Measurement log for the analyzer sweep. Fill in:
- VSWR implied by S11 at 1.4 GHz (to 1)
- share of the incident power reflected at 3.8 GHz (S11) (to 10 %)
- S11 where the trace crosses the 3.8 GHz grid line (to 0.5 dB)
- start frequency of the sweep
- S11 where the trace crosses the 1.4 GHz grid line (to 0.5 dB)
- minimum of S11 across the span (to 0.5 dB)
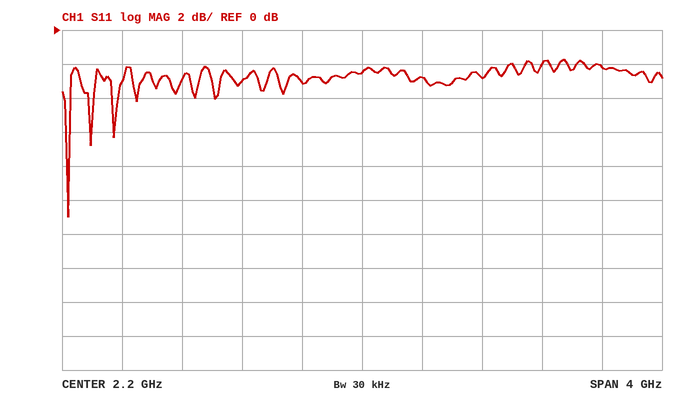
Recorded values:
6
60 %
-2.0 dB
200 MHz
-3.0 dB
-11.0 dB
